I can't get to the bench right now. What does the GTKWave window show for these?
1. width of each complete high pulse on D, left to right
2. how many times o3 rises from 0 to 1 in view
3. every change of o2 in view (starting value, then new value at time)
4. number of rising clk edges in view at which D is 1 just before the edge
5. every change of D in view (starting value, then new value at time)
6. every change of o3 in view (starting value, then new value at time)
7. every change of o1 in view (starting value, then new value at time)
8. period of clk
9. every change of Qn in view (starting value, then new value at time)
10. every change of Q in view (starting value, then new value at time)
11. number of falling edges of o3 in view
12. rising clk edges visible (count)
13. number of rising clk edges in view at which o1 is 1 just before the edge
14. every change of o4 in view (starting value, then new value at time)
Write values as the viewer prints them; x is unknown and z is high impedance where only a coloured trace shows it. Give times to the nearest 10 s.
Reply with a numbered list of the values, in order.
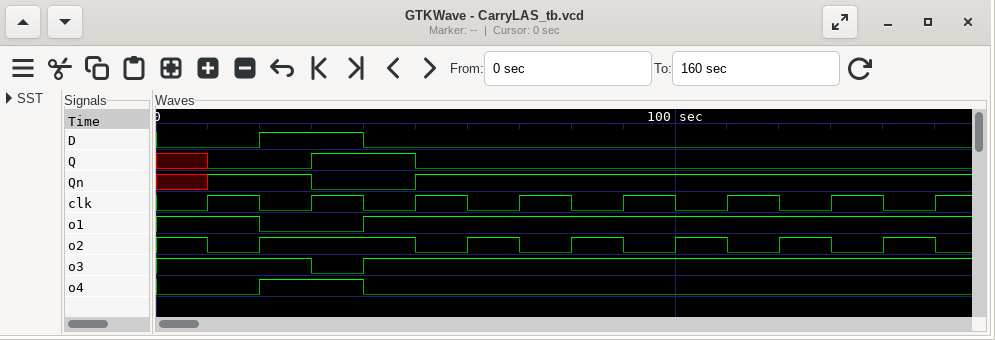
1. 20 s
2. 1
3. 1, 0 at 10 s, 1 at 20 s, 0 at 50 s, 1 at 60 s, 0 at 70 s, 1 at 80 s, 0 at 90 s, 1 at 100 s, 0 at 110 s, 1 at 120 s, 0 at 130 s, 1 at 140 s, 0 at 150 s
4. 1
5. 0, 1 at 20 s, 0 at 40 s
6. 1, 0 at 30 s, 1 at 40 s
7. 1, 0 at 20 s, 1 at 40 s
8. 20 s
9. x, 1 at 10 s, 0 at 30 s, 1 at 50 s
10. x, 0 at 10 s, 1 at 30 s, 0 at 50 s
11. 1
12. 8
13. 7
14. 0, 1 at 20 s, 0 at 40 s
